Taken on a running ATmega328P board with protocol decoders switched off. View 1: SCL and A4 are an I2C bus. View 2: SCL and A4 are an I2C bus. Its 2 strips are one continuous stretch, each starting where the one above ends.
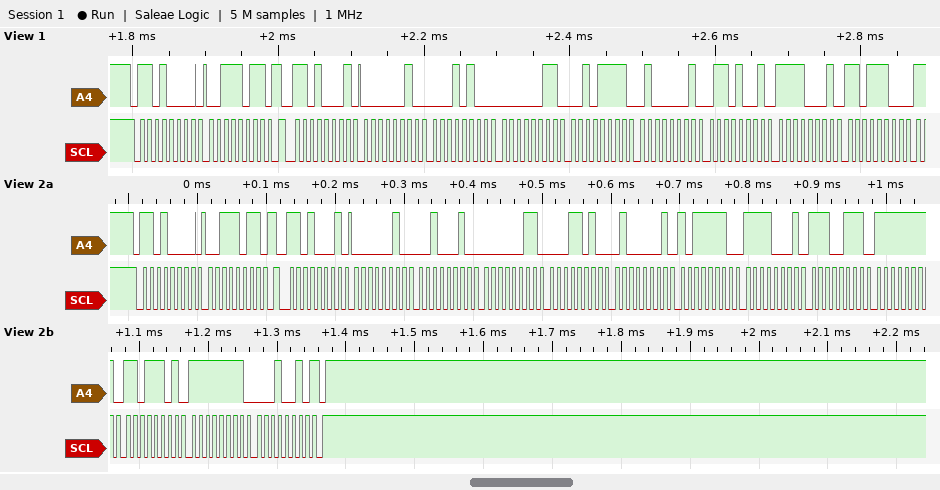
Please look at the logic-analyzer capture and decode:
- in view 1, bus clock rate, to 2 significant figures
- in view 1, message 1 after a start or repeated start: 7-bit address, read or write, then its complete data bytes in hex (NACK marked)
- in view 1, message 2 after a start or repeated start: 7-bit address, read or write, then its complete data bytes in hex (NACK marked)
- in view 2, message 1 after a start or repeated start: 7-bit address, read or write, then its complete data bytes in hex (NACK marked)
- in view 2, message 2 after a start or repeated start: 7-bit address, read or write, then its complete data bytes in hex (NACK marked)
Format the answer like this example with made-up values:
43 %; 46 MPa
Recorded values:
100 kHz; 0x68 write: 3B; 0x68 read: 02 14 03 2F 41 69 F1 DC; 0x68 write: 3B; 0x68 read: 02 22 03 1A 41 BE F1 E7 FF DD FF 12 NACK
